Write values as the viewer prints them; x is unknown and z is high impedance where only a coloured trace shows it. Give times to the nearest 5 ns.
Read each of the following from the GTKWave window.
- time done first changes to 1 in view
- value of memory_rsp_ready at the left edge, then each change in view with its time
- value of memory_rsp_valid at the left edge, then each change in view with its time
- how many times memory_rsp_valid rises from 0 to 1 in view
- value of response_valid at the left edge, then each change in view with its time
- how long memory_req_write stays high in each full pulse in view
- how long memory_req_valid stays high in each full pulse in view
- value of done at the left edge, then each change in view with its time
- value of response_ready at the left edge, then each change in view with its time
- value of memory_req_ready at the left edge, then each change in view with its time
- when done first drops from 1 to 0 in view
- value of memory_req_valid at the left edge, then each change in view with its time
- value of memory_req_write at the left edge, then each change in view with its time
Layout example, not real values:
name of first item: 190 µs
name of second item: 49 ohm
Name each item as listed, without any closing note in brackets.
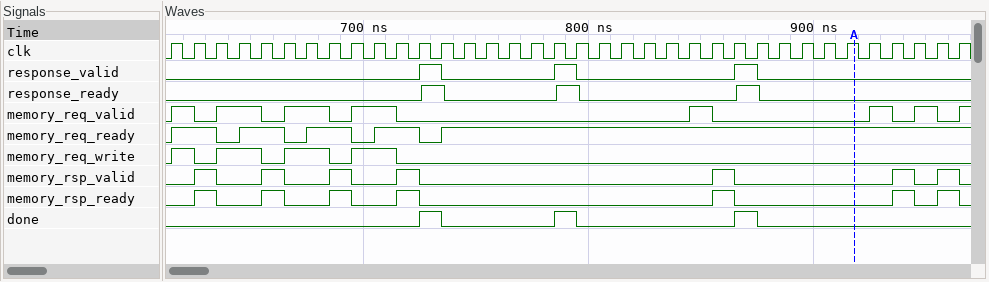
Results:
time done first changes to 1 in view: 725 ns
value of memory_rsp_ready at the left edge, then each change in view with its time: 0, 1 at 625 ns, 0 at 635 ns, 1 at 655 ns, 0 at 665 ns, 1 at 685 ns, 0 at 695 ns, 1 at 715 ns, 0 at 725 ns, 1 at 855 ns, 0 at 865 ns, 1 at 935 ns, 0 at 945 ns, 1 at 955 ns, 0 at 965 ns
value of memory_rsp_valid at the left edge, then each change in view with its time: 0, 1 at 625 ns, 0 at 635 ns, 1 at 655 ns, 0 at 665 ns, 1 at 685 ns, 0 at 695 ns, 1 at 715 ns, 0 at 725 ns, 1 at 855 ns, 0 at 865 ns, 1 at 935 ns, 0 at 945 ns, 1 at 955 ns, 0 at 965 ns
how many times memory_rsp_valid rises from 0 to 1 in view: 7
value of response_valid at the left edge, then each change in view with its time: 0, 1 at 725 ns, 0 at 735 ns, 1 at 785 ns, 0 at 795 ns, 1 at 865 ns, 0 at 875 ns
how long memory_req_write stays high in each full pulse in view: 10 ns, 20 ns, 20 ns, 20 ns
how long memory_req_valid stays high in each full pulse in view: 10 ns, 20 ns, 20 ns, 20 ns, 10 ns, 10 ns, 10 ns
value of done at the left edge, then each change in view with its time: 0, 1 at 725 ns, 0 at 735 ns, 1 at 785 ns, 0 at 795 ns, 1 at 865 ns, 0 at 875 ns
value of response_ready at the left edge, then each change in view with its time: 0, 1 at 725 ns, 0 at 735 ns, 1 at 785 ns, 0 at 795 ns, 1 at 865 ns, 0 at 875 ns
value of memory_req_ready at the left edge, then each change in view with its time: 0, 1 at 615 ns, 0 at 635 ns, 1 at 645 ns, 0 at 665 ns, 1 at 675 ns, 0 at 695 ns, 1 at 705 ns, 0 at 725 ns, 1 at 735 ns
when done first drops from 1 to 0 in view: 735 ns
value of memory_req_valid at the left edge, then each change in view with its time: 0, 1 at 615 ns, 0 at 625 ns, 1 at 635 ns, 0 at 655 ns, 1 at 665 ns, 0 at 685 ns, 1 at 695 ns, 0 at 715 ns, 1 at 845 ns, 0 at 855 ns, 1 at 925 ns, 0 at 935 ns, 1 at 945 ns, 0 at 955 ns, 1 at 965 ns
value of memory_req_write at the left edge, then each change in view with its time: 0, 1 at 615 ns, 0 at 625 ns, 1 at 635 ns, 0 at 655 ns, 1 at 665 ns, 0 at 685 ns, 1 at 695 ns, 0 at 715 ns
